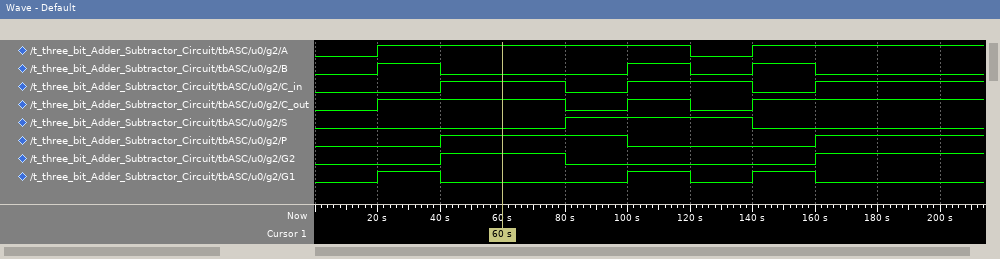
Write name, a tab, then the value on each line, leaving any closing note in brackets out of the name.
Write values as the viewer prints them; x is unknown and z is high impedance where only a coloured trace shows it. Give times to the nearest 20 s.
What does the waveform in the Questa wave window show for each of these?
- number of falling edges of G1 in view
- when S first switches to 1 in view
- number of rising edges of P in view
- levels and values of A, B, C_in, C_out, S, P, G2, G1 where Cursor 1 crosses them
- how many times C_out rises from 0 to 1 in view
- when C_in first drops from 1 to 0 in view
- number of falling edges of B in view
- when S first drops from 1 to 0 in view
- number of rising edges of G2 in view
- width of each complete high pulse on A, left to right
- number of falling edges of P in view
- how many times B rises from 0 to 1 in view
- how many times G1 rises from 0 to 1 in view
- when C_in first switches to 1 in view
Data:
number of falling edges of G1 in view	3
when S first switches to 1 in view	80 s
number of rising edges of P in view	2
levels and values of A, B, C_in, C_out, S, P, G2, G1 where Cursor 1 crosses them	A=1, B=0, C_in=1, C_out=1, S=0, P=1, G2=1, G1=0
how many times C_out rises from 0 to 1 in view	3
when C_in first drops from 1 to 0 in view	80 s
number of falling edges of B in view	3
when S first drops from 1 to 0 in view	140 s
number of rising edges of G2 in view	2
width of each complete high pulse on A, left to right	100 s
number of falling edges of P in view	1
how many times B rises from 0 to 1 in view	3
how many times G1 rises from 0 to 1 in view	3
when C_in first switches to 1 in view	40 s
